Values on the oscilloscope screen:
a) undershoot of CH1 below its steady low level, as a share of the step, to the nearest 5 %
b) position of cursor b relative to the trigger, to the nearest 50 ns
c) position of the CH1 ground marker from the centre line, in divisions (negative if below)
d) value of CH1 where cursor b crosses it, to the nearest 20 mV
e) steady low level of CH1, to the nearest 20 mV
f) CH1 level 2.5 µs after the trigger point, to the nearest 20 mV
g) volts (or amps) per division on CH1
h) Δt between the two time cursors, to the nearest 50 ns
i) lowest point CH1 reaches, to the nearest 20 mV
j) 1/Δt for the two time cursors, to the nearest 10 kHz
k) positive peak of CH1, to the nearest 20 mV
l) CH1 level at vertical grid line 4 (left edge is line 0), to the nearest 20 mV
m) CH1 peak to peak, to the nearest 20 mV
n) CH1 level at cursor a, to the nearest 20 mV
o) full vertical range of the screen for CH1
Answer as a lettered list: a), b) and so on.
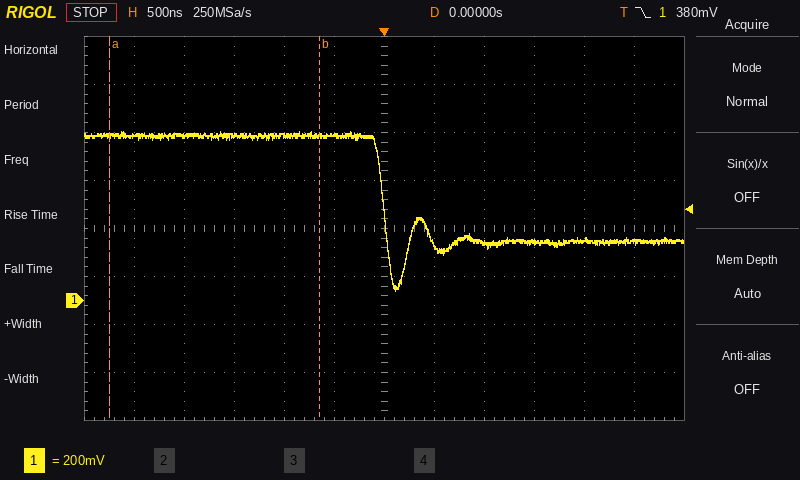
a) 45 %
b) -650 ns
c) -1.5 div
d) 680 mV
e) 240 mV
f) 240 mV
g) 200 mV
h) 2.10 µs
i) 40 mV
j) 480 kHz
k) 700 mV
l) 680 mV
m) 660 mV
n) 680 mV
o) 1.6 V
